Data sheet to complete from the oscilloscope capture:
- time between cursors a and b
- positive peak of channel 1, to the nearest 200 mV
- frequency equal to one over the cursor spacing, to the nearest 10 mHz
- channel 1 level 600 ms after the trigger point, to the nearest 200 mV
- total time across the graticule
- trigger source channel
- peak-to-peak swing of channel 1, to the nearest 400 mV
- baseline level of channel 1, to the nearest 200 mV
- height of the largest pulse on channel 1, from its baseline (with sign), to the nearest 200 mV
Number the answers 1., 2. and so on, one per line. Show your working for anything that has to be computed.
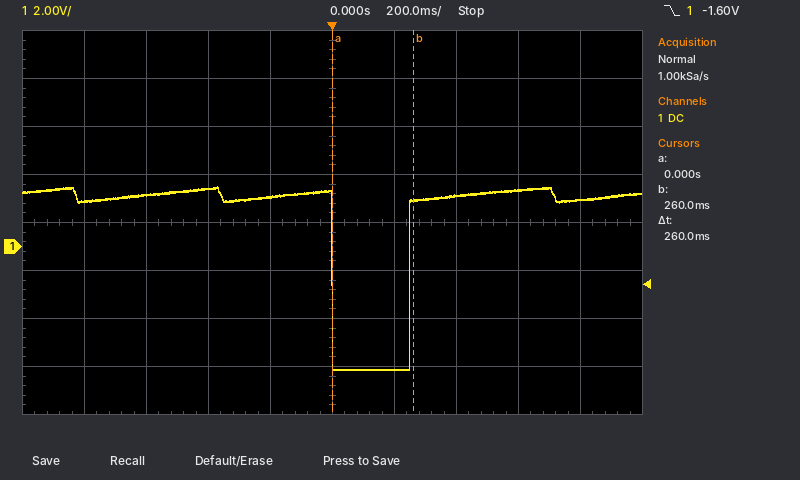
1. 260 ms
2. 2.4 V
3. 1 / 260 ms ≈ 3.85 Hz
4. 2.4 V
5. 2 s
6. channel 1
7. 7.6 V
8. 2.2 V
9. -7.2 V
